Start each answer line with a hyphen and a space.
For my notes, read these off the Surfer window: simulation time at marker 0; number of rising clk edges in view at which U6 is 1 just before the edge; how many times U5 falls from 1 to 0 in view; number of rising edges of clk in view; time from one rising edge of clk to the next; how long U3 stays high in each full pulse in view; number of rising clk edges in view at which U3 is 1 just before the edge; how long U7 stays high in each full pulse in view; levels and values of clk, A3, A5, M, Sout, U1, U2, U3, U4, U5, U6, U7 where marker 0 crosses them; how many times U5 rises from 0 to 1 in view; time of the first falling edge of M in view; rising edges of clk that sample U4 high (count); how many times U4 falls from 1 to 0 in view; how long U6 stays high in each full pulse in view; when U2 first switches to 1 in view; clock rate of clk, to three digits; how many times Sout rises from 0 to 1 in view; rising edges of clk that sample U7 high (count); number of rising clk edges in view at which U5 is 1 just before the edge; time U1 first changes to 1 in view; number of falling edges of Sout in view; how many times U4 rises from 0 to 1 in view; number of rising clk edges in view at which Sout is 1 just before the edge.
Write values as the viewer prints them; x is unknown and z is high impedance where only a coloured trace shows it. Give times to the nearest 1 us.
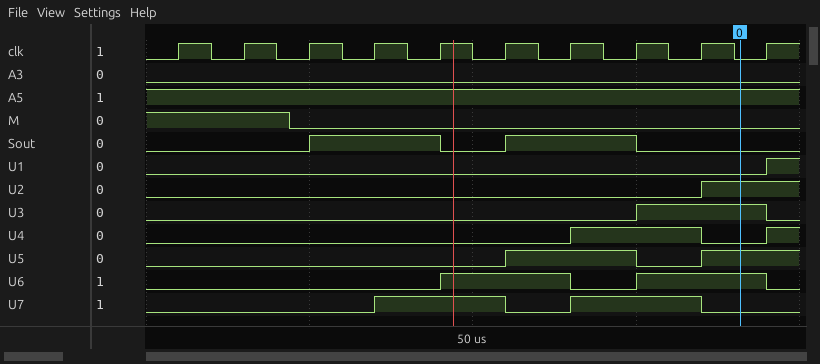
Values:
- 91 us
- 4
- 1
- 10
- 10 us
- 20 us
- 2
- 20 us, 20 us
- clk=0, A3=0, A5=1, M=0, Sout=0, U1=0, U2=1, U3=1, U4=0, U5=1, U6=1, U7=0
- 2
- 22 us
- 2
- 1
- 20 us, 20 us
- 85 us
- 100 kHz
- 2
- 4
- 3
- 95 us
- 2
- 2
- 4
